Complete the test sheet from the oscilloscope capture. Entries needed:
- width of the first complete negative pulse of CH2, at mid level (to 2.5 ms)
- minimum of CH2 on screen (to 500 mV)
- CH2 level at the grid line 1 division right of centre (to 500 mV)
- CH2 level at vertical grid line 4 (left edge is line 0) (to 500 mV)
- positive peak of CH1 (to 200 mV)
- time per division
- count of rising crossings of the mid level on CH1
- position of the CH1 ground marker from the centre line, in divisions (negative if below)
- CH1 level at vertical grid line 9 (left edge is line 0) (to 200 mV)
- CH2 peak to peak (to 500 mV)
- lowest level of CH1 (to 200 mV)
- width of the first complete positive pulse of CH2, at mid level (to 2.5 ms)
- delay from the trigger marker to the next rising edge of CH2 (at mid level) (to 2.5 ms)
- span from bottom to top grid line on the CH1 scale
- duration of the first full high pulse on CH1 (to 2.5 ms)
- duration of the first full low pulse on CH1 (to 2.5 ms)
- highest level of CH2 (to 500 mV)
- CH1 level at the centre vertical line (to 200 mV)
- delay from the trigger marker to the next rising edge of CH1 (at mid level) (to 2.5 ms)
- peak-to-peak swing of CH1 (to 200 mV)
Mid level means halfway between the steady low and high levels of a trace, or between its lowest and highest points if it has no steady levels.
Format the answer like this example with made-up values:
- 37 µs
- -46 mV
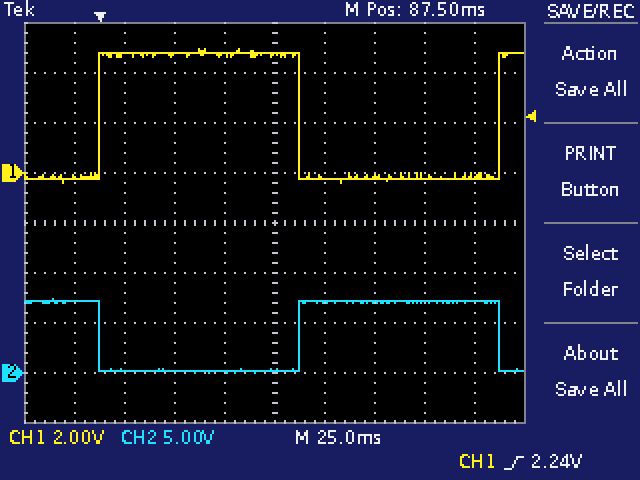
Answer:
- 100.0 ms
- 0.0 V
- 7.0 V
- 0.0 V
- 5.0 V
- 25 ms
- 2
- +1.0 div
- -200 mV
- 7.5 V
- -400 mV
- 100.0 ms
- 100.0 ms
- 16 V
- 100.0 ms
- 100.0 ms
- 7.5 V
- 4.8 V
- 200.0 ms
- 5.4 V
